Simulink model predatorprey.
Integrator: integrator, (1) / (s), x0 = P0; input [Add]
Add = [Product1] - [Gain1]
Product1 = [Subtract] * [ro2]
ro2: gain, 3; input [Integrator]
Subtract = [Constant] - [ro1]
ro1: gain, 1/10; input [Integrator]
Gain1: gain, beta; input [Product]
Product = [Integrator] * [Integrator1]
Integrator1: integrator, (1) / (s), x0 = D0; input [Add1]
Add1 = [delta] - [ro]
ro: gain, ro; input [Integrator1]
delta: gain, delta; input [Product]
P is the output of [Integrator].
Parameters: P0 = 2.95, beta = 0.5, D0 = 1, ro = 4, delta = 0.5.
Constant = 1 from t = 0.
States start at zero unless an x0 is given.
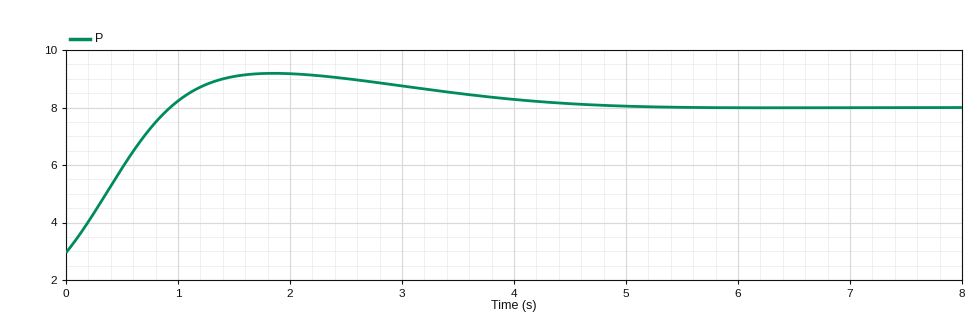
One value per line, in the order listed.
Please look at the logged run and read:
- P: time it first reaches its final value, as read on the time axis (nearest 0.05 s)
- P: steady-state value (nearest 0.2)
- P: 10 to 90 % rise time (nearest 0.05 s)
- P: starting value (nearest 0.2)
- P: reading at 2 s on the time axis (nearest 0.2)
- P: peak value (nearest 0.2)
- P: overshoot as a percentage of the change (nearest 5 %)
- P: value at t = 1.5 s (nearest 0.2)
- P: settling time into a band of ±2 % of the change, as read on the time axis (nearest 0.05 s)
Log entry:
0.95 s
8.0
0.70 s
3.0
9.2
9.2
25 %
9.0
4.65 s
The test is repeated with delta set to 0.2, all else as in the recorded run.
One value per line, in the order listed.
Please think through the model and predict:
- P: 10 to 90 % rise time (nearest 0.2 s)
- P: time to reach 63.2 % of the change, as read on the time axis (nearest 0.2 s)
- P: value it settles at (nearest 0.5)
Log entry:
1.2 s
0.8 s
10.0
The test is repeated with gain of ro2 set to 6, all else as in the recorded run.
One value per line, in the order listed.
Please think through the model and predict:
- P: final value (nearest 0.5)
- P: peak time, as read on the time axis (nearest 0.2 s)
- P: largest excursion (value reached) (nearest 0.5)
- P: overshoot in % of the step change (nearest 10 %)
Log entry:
8.0
1.0 s
9.5
30 %
